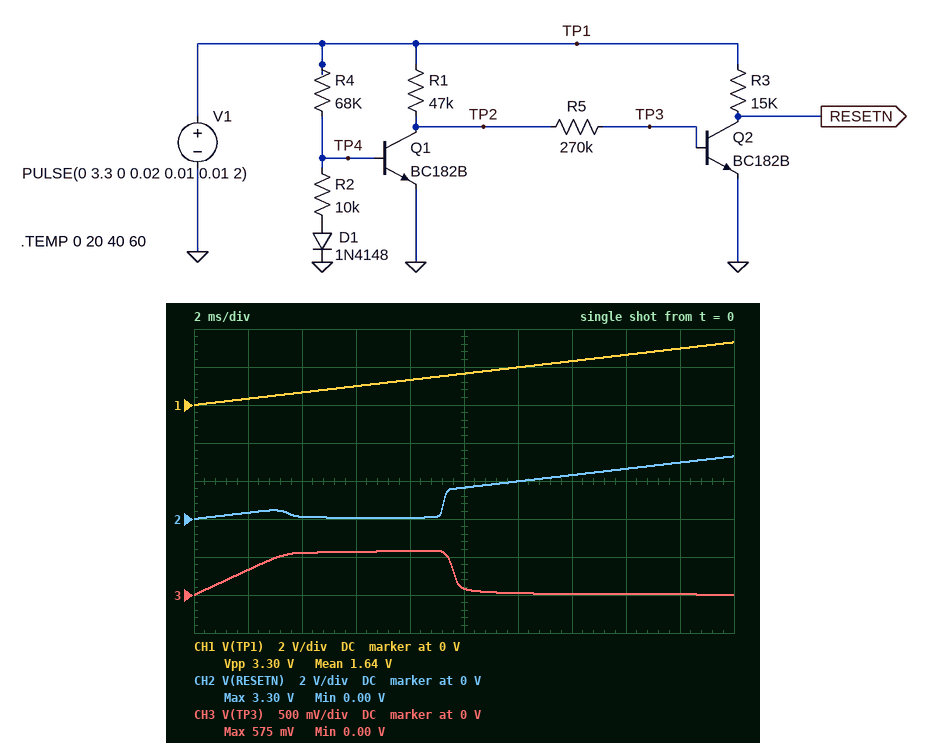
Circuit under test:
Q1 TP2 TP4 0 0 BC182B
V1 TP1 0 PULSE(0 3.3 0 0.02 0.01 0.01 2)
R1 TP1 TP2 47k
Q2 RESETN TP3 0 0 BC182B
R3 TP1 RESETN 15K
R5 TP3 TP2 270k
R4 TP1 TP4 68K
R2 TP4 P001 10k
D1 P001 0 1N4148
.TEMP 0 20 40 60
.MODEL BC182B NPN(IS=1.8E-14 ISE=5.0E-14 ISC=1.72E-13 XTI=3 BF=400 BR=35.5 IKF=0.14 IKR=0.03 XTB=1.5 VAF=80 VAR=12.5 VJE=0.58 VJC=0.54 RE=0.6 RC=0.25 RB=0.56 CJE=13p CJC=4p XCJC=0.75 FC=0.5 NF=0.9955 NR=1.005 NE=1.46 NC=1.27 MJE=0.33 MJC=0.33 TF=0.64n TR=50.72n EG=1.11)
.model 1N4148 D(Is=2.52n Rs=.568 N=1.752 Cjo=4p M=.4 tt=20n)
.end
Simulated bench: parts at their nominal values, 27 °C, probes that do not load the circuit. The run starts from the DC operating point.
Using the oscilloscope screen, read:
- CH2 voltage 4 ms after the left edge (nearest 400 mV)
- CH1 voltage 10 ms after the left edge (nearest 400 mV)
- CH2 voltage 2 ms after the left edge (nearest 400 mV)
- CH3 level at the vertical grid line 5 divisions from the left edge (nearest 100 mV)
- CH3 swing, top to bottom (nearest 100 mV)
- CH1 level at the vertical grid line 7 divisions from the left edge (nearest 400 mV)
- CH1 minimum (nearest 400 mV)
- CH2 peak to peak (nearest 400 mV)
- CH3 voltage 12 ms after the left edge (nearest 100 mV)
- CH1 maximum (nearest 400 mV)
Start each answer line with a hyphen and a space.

- 0 V
- 1.6 V
- 400 mV
- 100 mV
- 600 mV
- 2.4 V
- 0 V
- 3.2 V
- 0 V
- 3.2 V
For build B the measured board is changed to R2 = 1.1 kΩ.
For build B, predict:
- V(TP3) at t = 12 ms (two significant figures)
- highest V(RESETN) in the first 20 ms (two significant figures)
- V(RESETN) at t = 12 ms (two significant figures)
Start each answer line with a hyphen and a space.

- 590 mV
- 460 mV
- 44 mV
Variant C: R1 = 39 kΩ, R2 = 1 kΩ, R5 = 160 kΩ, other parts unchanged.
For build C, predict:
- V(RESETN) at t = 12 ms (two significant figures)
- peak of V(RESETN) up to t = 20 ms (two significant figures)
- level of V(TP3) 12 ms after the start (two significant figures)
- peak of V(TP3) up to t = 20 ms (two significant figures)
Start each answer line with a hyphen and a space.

- 31 mV
- 450 mV
- 590 mV
- 610 mV
